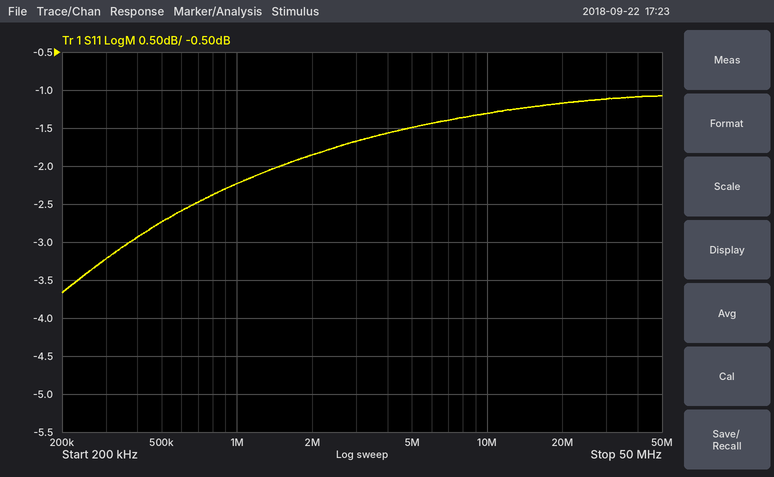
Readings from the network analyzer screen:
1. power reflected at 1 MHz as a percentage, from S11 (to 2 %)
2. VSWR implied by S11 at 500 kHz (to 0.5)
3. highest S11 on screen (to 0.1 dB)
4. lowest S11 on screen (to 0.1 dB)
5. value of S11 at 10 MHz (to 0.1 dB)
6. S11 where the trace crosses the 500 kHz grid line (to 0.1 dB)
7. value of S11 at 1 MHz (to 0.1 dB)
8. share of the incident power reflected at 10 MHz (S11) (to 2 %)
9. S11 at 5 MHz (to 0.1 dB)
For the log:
60 %
6.5
-1.1 dB
-3.7 dB
-1.3 dB
-2.7 dB
-2.2 dB
74 %
-1.5 dB
